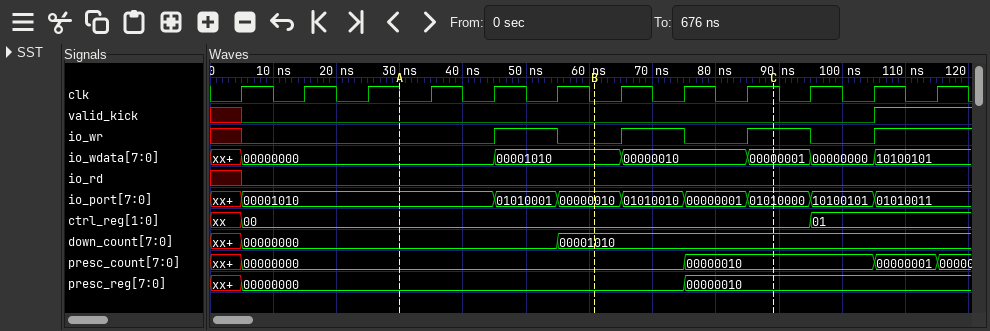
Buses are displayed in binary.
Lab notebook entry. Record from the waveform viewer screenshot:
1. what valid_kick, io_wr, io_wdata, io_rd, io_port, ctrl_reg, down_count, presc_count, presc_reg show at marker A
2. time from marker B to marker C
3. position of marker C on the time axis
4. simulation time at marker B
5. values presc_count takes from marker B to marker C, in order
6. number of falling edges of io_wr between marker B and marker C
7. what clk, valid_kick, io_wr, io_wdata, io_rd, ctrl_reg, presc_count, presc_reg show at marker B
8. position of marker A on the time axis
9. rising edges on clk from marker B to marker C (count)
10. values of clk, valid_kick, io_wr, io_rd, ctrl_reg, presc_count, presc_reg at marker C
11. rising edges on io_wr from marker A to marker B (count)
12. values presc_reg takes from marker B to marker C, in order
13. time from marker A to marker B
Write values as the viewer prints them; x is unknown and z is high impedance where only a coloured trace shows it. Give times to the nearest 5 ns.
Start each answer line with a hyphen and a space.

- valid_kick=0, io_wr=0, io_wdata=00000000, io_rd=0, io_port=00001010, ctrl_reg=00, down_count=00000000, presc_count=00000000, presc_reg=00000000
- 30 ns
- 90 ns
- 60 ns
- 00000000, 00000010
- 1
- clk=0, valid_kick=0, io_wr=0, io_wdata=00001010, io_rd=0, ctrl_reg=00, presc_count=00000000, presc_reg=00000000
- 30 ns
- 3
- clk=1, valid_kick=0, io_wr=1, io_rd=0, ctrl_reg=00, presc_count=00000010, presc_reg=00000010
- 1
- 00000000, 00000010
- 30 ns
